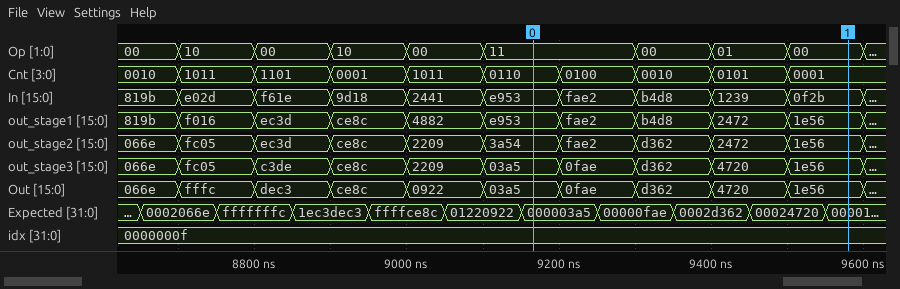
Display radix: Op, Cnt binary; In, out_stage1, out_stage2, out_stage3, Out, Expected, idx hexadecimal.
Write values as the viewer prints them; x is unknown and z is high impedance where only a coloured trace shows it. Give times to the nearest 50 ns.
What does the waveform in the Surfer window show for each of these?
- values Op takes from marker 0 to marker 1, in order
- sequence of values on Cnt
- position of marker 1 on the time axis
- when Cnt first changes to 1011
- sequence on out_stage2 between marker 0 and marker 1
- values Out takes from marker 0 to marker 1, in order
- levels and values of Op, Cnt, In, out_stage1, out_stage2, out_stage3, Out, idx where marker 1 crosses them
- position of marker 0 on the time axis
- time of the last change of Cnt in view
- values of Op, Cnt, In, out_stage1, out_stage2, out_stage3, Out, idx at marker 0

11, 00, 01, 00
0010, 1011, 1101, 0001, 1011, 0110, 0100, 0010, 0101, 0001
9600 ns
8700 ns
3a54, fae2, d362, 2472, 1e56
03a5, 0fae, d362, 4720, 1e56
Op=00, Cnt=0001, In=0f2b, out_stage1=1e56, out_stage2=1e56, out_stage3=1e56, Out=1e56, idx=0000000f
9150 ns
9500 ns
Op=11, Cnt=0110, In=e953, out_stage1=e953, out_stage2=3a54, out_stage3=03a5, Out=03a5, idx=0000000f
